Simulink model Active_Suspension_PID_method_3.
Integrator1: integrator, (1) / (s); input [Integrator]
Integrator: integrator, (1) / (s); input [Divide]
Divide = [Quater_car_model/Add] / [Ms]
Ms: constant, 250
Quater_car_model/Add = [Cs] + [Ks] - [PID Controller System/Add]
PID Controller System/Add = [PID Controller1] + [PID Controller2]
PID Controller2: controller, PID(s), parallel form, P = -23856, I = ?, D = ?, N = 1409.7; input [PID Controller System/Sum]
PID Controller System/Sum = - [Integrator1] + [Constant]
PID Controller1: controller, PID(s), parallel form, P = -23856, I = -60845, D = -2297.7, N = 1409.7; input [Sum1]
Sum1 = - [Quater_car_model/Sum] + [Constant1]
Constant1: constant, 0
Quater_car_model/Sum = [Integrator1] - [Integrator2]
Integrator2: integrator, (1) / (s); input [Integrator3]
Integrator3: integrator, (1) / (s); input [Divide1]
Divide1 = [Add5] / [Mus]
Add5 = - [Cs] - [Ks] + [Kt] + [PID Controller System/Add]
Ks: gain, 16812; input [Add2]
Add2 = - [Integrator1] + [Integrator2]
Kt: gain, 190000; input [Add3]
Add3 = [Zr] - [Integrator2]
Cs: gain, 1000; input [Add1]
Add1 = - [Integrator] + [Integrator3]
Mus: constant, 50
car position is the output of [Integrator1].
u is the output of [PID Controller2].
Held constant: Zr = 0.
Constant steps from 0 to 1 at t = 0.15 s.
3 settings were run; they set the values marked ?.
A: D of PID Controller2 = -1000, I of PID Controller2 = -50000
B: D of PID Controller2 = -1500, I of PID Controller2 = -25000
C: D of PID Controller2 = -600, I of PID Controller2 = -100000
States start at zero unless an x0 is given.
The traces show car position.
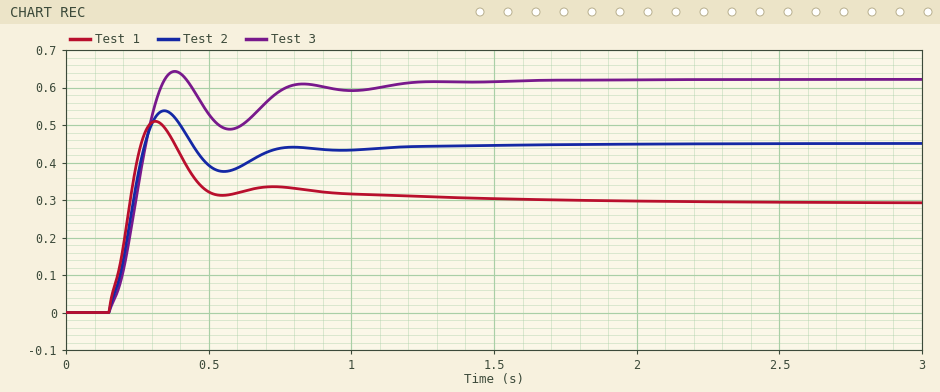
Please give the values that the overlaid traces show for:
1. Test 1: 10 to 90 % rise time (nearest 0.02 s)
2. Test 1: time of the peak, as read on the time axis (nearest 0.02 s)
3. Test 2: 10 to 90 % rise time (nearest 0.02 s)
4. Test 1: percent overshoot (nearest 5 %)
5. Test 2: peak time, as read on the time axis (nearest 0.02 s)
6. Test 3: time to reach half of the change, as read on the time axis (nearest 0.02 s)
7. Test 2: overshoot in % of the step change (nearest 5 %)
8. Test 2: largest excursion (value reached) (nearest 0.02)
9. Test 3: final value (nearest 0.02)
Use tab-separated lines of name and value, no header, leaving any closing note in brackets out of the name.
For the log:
Test 1: 10 to 90 % rise time	0.06 s
Test 1: time of the peak, as read on the time axis	0.32 s
Test 2: 10 to 90 % rise time	0.10 s
Test 1: percent overshoot	75 %
Test 2: peak time, as read on the time axis	0.34 s
Test 3: time to reach half of the change, as read on the time axis	0.24 s
Test 2: overshoot in % of the step change	20 %
Test 2: largest excursion (value reached)	0.54
Test 3: final value	0.62
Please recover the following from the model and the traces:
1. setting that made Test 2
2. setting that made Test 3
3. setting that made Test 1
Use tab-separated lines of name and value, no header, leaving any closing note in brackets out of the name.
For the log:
setting that made Test 2	A
setting that made Test 3	C
setting that made Test 1	B
